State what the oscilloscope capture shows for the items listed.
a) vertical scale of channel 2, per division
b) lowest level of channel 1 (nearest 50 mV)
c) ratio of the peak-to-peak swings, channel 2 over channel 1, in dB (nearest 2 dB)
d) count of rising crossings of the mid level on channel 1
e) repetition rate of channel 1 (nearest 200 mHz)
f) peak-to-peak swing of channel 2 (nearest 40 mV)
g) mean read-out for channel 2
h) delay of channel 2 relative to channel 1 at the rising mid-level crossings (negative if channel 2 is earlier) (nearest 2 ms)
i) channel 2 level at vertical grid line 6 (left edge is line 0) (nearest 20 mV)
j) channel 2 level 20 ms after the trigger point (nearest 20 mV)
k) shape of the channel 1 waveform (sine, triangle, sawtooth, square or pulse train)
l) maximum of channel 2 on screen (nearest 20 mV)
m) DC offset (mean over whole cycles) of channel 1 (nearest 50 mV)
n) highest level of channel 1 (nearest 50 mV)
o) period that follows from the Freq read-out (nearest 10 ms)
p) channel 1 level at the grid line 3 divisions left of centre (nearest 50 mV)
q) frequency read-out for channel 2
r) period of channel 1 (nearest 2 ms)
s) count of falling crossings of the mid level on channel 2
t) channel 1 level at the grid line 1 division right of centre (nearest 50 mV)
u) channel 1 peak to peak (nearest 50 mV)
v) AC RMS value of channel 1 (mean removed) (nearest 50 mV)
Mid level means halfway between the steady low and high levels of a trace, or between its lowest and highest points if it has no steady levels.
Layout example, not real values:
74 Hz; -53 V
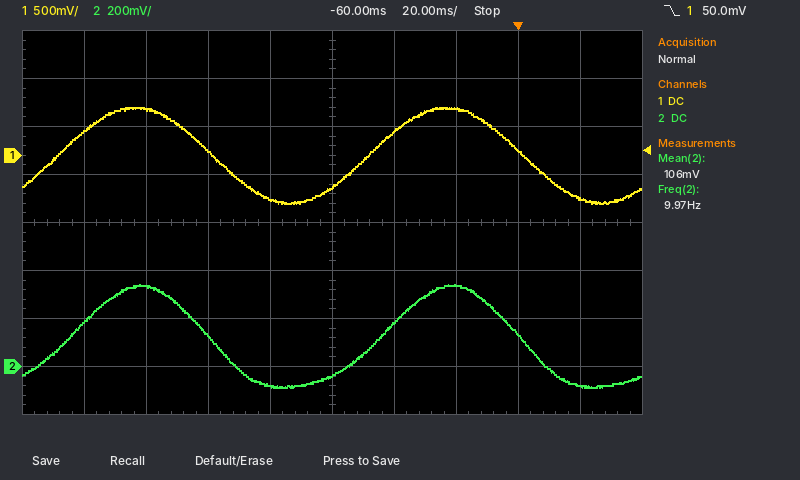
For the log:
200 mV; -500 mV; -8 dB; 2; 10.0 Hz; 440 mV; 106 mV; +4 ms; 180 mV; -80 mV; sine; 340 mV; 0 mV; 500 mV; 100 ms; 500 mV; 9.97 Hz; 100 ms; 2; 250 mV; 1.00 V; 350 mV
